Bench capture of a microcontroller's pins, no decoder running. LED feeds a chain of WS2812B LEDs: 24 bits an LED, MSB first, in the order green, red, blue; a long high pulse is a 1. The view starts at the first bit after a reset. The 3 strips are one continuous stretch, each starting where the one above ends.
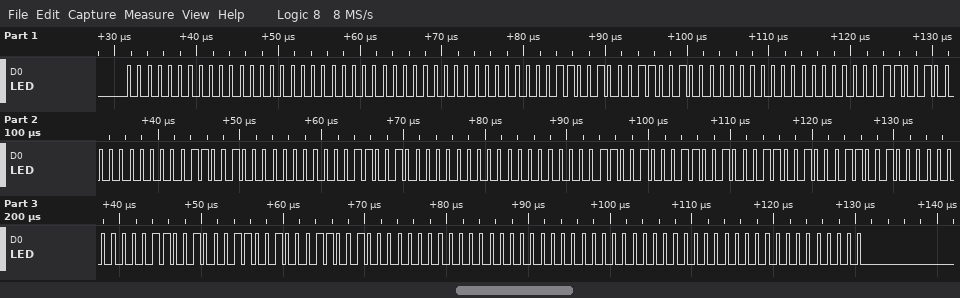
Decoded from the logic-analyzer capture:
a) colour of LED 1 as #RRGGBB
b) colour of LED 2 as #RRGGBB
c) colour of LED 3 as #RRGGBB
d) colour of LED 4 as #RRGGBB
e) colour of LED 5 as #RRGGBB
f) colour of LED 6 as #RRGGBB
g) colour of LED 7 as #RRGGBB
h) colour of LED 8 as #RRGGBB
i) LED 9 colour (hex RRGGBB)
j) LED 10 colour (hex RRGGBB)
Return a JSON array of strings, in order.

["#000000", "#000032", "#003200", "#003232", "#320000", "#320032", "#323200", "#323232", "#000000", "#000000"]
